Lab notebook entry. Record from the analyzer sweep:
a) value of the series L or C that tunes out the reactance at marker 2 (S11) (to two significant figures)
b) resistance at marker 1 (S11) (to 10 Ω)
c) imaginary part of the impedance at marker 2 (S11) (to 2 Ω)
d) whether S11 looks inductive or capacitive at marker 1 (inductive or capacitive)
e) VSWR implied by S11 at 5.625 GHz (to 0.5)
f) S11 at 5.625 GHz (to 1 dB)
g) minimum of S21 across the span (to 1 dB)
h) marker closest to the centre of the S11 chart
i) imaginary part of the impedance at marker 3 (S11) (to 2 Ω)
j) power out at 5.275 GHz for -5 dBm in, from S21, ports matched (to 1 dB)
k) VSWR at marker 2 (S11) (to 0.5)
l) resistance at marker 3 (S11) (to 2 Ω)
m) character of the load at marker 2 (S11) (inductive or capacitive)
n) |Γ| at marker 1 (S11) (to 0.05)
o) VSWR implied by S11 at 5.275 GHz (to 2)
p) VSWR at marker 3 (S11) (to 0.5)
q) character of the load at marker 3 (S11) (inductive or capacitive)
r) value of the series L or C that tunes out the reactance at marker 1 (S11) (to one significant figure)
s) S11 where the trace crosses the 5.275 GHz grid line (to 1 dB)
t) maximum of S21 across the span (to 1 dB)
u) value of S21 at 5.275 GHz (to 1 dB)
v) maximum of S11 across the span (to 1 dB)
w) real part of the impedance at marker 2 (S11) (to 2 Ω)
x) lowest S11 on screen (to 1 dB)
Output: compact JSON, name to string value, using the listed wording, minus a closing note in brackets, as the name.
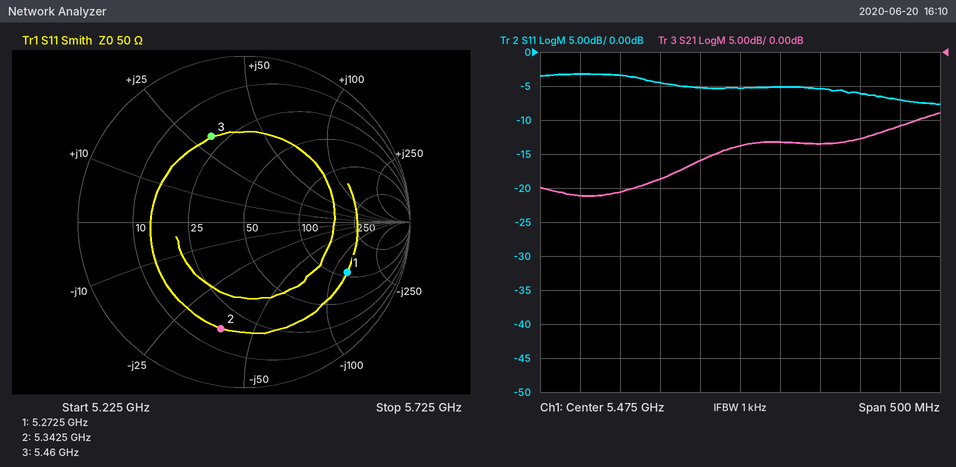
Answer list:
{"value of the series L or C that tunes out the reactance at marker 2 (S11)": "1.1 nH", "resistance at marker 1 (S11)": "110 Ω", "imaginary part of the impedance at marker 2 (S11)": "-38 Ω", "whether S11 looks inductive or capacitive at marker 1": "capacitive", "VSWR implied by S11 at 5.625 GHz": "3.0", "S11 at 5.625 GHz": "-6 dB", "minimum of S21 across the span": "-21 dB", "marker closest to the centre of the S11 chart": "marker 3", "imaginary part of the impedance at marker 3 (S11)": "+30 Ω", "power out at 5.275 GHz for -5 dBm in, from S21, ports matched": "-26 dBm", "VSWR at marker 2 (S11)": "5.0", "resistance at marker 3 (S11)": "20 Ω", "character of the load at marker 2 (S11)": "capacitive", "|Γ| at marker 1 (S11)": "0.70", "VSWR implied by S11 at 5.275 GHz": "6", "VSWR at marker 3 (S11)": "3.5", "character of the load at marker 3 (S11)": "inductive", "value of the series L or C that tunes out the reactance at marker 1 (S11)": "4 nH", "S11 where the trace crosses the 5.275 GHz grid line": "-3 dB", "maximum of S21 across the span": "-9 dB", "value of S21 at 5.275 GHz": "-21 dB", "maximum of S11 across the span": "-3 dB", "real part of the impedance at marker 2 (S11)": "16 Ω", "lowest S11 on screen": "-8 dB"}
